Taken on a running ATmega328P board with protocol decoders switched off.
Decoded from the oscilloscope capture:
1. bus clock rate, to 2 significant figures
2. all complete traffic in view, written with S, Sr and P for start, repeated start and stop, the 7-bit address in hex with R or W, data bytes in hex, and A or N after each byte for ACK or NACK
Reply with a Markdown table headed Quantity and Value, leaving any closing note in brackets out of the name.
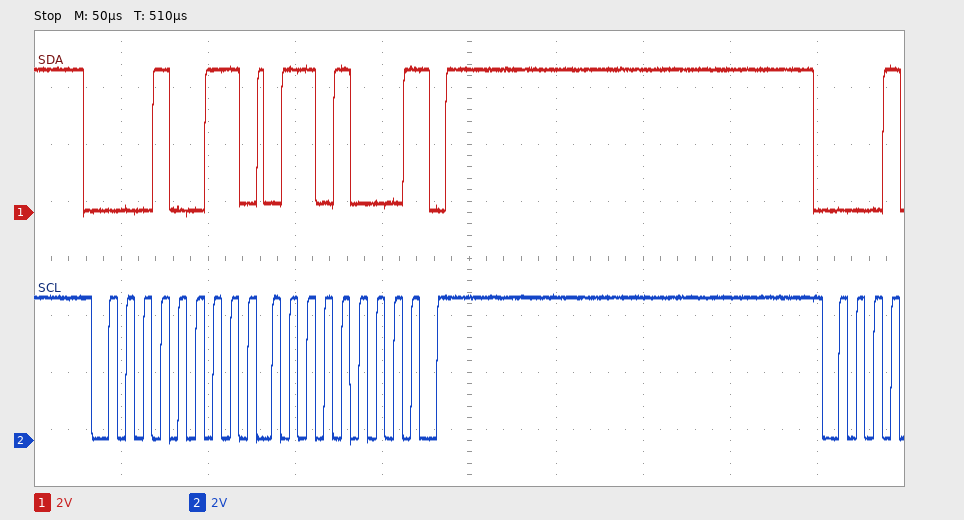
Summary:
| Quantity | Value |
|---|---|
| bus clock rate, to 2 significant figures | 100 kHz |
| all complete traffic in view, written with S, Sr and P for start, repeated start and stop, the 7-bit address in hex with R or W, data bytes in hex, and A or N after each byte for ACK or NACK | S 09R A 68 N P |
